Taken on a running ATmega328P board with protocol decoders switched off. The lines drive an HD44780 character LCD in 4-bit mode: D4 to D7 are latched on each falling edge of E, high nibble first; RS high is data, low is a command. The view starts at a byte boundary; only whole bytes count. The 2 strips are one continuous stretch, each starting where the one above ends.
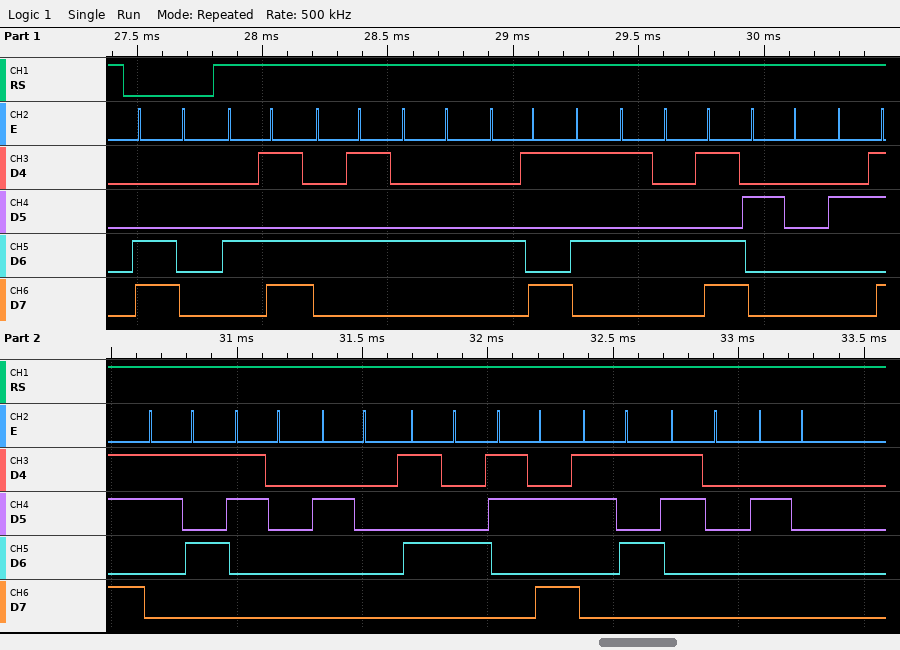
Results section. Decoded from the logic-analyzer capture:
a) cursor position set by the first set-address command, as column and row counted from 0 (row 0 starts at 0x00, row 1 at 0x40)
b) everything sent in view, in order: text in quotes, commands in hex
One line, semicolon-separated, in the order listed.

column 0, row 1; 0xC0 "MEDIUM +50 T:50 "
